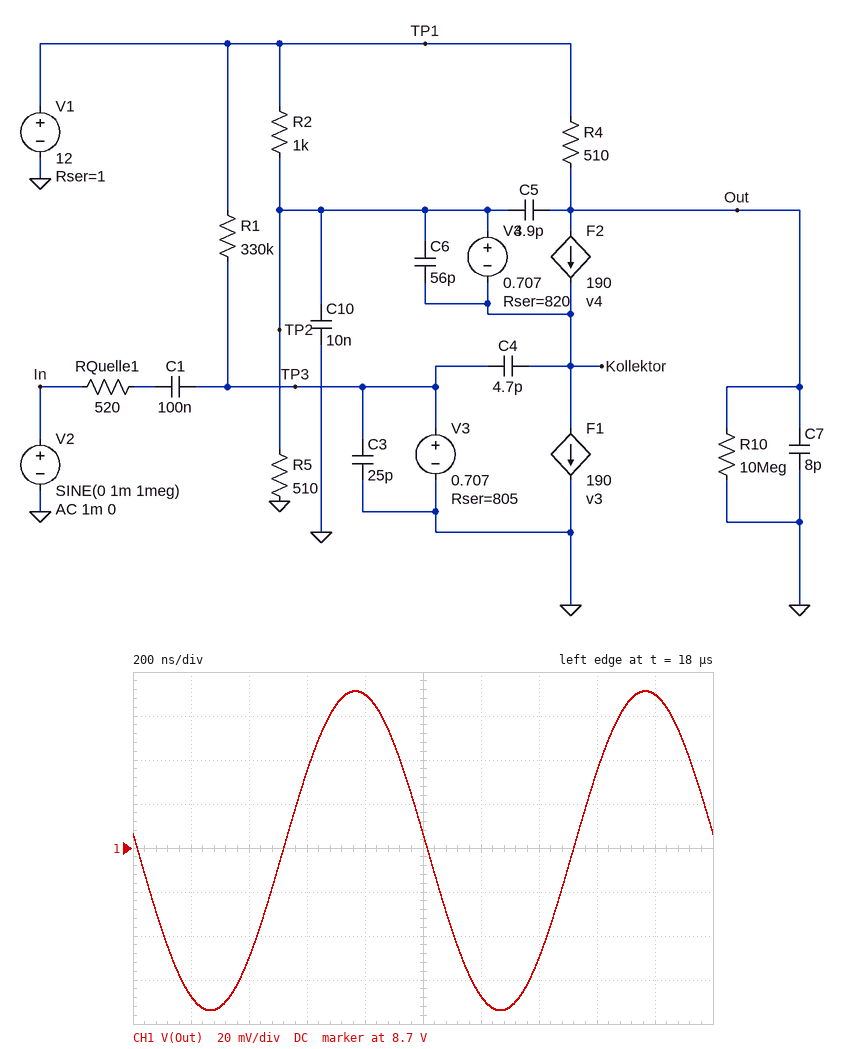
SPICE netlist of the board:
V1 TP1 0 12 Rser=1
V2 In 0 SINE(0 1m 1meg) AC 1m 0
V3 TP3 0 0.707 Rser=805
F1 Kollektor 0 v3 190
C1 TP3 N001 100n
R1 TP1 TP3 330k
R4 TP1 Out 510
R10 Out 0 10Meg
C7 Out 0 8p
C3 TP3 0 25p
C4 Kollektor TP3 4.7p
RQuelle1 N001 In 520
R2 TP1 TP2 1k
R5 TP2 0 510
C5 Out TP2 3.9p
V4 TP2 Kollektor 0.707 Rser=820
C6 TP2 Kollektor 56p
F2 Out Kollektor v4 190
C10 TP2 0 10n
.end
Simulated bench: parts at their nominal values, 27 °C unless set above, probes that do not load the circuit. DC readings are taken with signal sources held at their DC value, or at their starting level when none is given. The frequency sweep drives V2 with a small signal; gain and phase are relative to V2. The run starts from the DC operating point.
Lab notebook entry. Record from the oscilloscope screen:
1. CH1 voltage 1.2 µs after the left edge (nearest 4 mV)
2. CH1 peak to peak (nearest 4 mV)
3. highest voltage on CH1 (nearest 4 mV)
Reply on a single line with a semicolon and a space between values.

8.632 V; 144 mV; 8.772 V
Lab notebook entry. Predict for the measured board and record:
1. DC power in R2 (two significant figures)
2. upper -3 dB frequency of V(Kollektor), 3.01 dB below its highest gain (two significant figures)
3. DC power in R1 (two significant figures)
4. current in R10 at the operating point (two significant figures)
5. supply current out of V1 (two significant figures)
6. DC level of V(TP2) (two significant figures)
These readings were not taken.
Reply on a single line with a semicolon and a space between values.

63 mW; 2.6 MHz; 380 µW; 870 nA; 14 mA; 4.0 V
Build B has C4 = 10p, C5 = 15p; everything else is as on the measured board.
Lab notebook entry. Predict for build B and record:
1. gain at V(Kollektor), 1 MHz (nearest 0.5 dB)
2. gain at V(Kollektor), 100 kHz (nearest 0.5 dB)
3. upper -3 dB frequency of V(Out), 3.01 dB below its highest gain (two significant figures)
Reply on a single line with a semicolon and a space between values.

-3.0 dB; -2.5 dB; 7.6 MHz
